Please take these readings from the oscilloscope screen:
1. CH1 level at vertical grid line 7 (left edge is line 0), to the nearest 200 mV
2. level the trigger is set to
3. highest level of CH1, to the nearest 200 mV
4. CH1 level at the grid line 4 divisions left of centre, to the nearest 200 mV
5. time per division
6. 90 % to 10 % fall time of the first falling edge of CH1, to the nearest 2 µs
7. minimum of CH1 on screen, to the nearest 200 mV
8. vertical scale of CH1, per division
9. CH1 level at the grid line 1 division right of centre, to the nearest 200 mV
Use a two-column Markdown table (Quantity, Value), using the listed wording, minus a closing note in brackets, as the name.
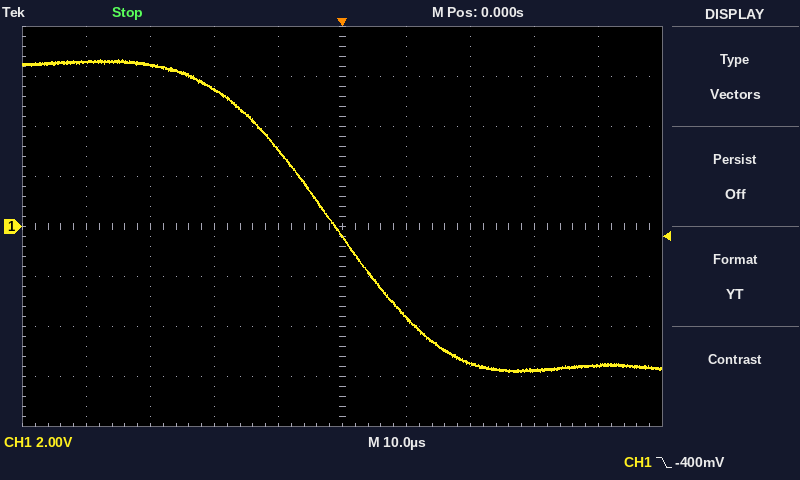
| Quantity | Value |
|---|---|
| CH1 level at vertical grid line 7 (left edge is line 0), to the nearest 200 mV | -5.4 V |
| level the trigger is set to | -400 mV |
| highest level of CH1, to the nearest 200 mV | 6.6 V |
| CH1 level at the grid line 4 divisions left of centre, to the nearest 200 mV | 6.6 V |
| time per division | 10 µs |
| 90 % to 10 % fall time of the first falling edge of CH1, to the nearest 2 µs | 32 µs |
| minimum of CH1 on screen, to the nearest 200 mV | -5.8 V |
| vertical scale of CH1, per division | 2 V |
| CH1 level at the grid line 1 division right of centre, to the nearest 200 mV | -3.6 V |
